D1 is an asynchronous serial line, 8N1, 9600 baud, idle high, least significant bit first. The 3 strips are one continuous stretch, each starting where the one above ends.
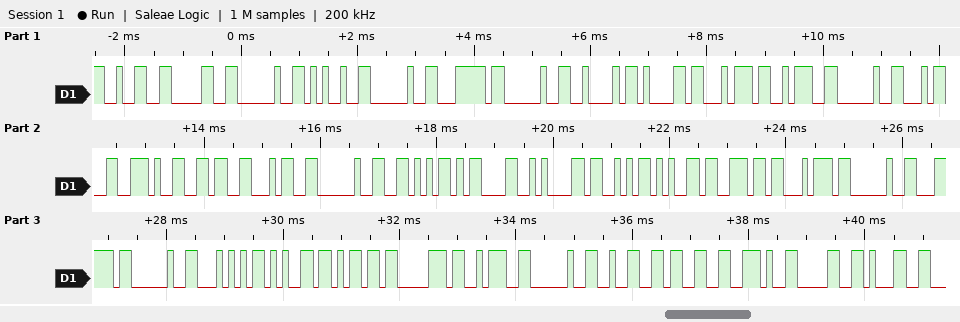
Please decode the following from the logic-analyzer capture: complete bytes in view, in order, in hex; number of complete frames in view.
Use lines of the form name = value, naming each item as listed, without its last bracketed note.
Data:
complete bytes in view, in order, in hex = 32 30 20 25 20 7C 20 42 61 74 3A 20 34 2E 36 34 20 56 0D 0A 53 65 6E 74 20 7C 20 54 65 6D 70 3A 20 32 33 2E 30 31
number of complete frames in view = 38
